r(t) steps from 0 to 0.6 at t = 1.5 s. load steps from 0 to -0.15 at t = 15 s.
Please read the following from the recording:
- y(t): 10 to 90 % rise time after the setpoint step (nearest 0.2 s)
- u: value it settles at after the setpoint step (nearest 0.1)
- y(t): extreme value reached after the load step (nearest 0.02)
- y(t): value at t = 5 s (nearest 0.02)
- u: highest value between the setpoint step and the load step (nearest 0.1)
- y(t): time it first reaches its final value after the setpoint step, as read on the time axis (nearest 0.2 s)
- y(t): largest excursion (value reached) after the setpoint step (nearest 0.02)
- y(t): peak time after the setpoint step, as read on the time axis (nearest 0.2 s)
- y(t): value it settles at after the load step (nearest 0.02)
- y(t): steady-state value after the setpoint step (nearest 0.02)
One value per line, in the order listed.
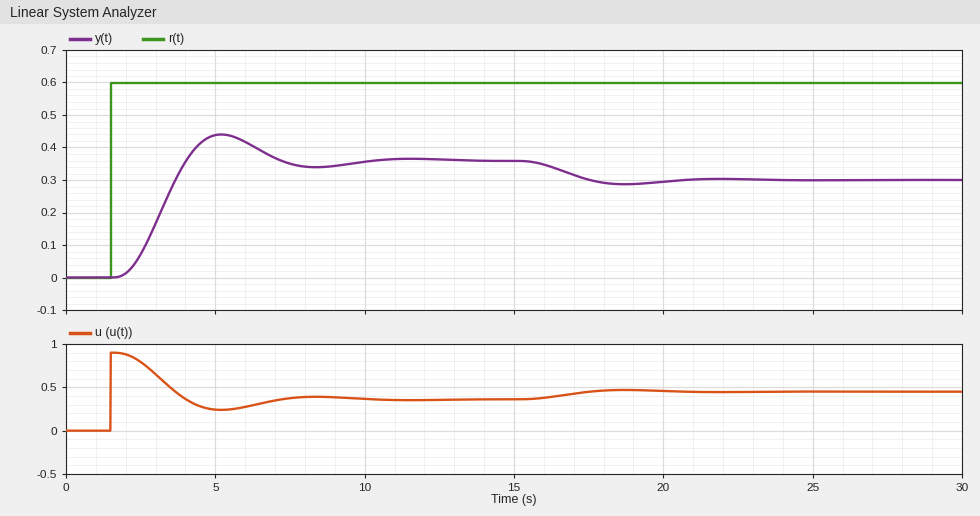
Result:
1.6 s
0.4
0.28
0.44
0.9
4.0 s
0.44
5.2 s
0.30
0.36
